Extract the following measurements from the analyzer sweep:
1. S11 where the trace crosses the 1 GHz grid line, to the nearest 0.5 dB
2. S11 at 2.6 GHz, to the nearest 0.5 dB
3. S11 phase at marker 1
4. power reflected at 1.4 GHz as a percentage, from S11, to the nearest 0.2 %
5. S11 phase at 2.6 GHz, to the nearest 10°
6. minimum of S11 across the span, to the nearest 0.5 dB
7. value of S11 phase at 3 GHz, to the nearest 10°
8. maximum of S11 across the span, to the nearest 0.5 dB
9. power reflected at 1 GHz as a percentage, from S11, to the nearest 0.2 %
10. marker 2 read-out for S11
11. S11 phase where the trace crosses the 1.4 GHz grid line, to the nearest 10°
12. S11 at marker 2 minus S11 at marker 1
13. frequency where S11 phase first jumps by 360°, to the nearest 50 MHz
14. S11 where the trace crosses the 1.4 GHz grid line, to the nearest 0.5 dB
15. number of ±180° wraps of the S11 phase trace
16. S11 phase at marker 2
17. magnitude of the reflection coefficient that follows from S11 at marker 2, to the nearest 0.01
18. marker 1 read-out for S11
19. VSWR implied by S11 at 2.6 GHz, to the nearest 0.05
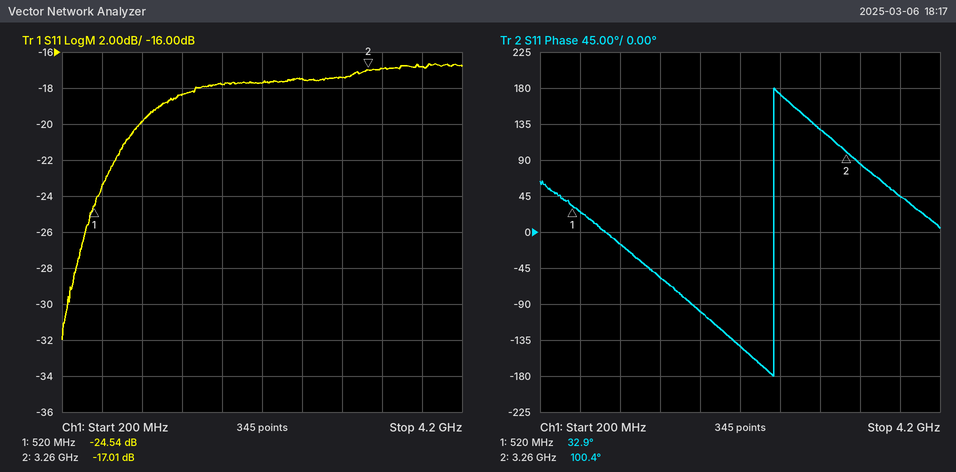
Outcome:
-20.0 dB
-17.5 dB
32.9°
1.4 %
170°
-32.0 dB
130°
-16.5 dB
1.0 %
-17.01 dB
-60°
7.53 dB
2.55 GHz
-18.5 dB
1
100.4°
0.14
-24.54 dB
1.30
